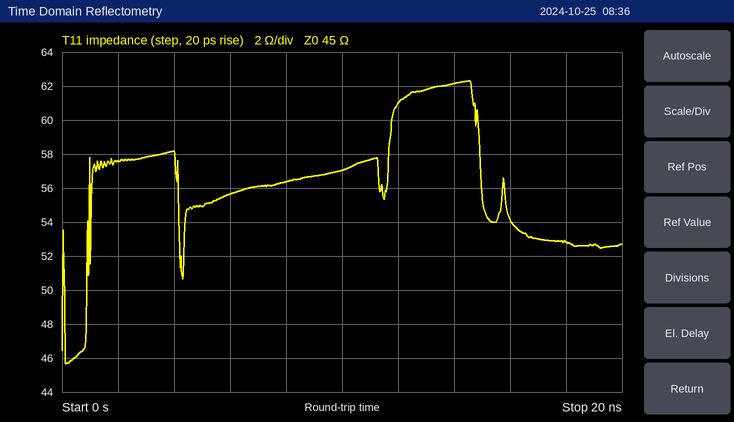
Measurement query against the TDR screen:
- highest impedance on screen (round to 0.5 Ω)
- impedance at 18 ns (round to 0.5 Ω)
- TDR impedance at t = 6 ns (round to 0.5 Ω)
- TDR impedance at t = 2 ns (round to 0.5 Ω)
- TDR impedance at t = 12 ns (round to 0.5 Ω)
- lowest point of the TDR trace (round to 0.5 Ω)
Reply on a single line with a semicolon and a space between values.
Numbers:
62.5 Ω; 53.0 Ω; 55.5 Ω; 57.5 Ω; 61.0 Ω; 45.5 Ω
